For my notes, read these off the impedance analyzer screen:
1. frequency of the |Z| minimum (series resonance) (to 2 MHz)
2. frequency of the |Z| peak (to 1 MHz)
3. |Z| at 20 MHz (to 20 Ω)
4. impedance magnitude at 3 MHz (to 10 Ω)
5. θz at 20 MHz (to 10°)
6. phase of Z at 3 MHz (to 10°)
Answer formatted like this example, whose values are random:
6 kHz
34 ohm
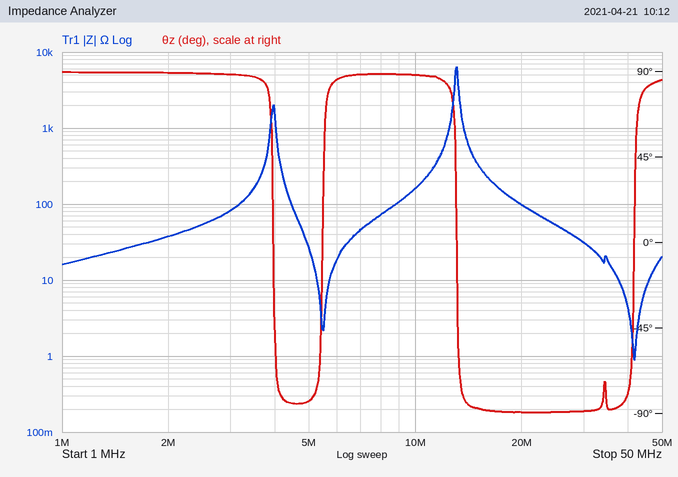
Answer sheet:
42 MHz
13 MHz
100 Ω
80 Ω
-90°
90°
